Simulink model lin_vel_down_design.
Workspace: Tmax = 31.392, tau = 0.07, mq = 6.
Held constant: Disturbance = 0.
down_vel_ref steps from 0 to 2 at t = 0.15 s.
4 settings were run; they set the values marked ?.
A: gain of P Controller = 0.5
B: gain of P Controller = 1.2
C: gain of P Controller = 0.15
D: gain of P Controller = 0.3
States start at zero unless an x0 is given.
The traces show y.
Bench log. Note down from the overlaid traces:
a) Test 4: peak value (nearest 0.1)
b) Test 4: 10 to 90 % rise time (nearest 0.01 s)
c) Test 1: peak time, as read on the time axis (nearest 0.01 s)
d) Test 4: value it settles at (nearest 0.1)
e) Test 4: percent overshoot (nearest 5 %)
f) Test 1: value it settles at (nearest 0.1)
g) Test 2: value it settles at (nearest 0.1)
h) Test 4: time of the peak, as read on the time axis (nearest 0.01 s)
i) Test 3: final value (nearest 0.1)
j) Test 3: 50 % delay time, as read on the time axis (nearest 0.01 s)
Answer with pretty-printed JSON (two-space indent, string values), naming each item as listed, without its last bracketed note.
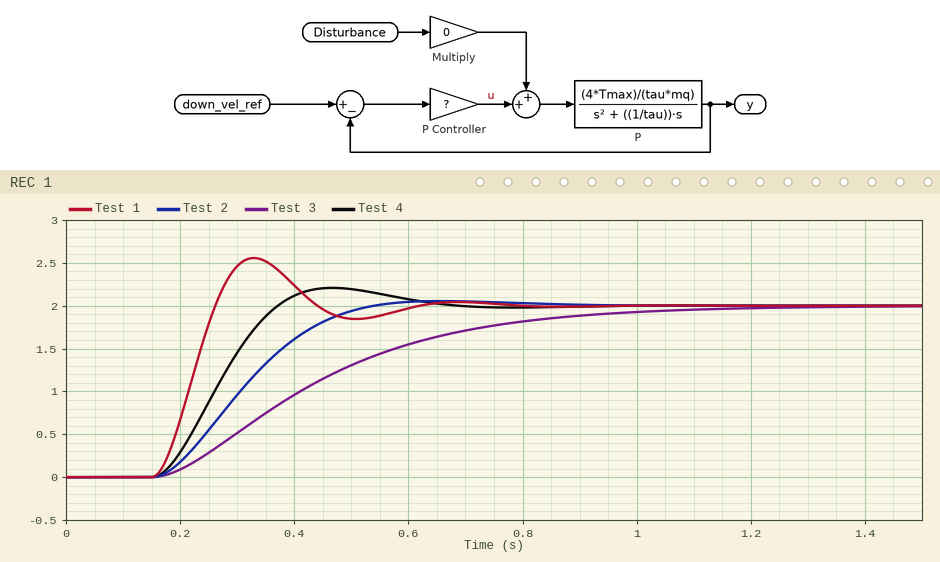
{
  "Test 4: peak value": "2.2",
  "Test 4: 10 to 90 % rise time": "0.15 s",
  "Test 1: peak time, as read on the time axis": "0.33 s",
  "Test 4: value it settles at": "2.0",
  "Test 4: percent overshoot": "10 %",
  "Test 1: value it settles at": "2.0",
  "Test 2: value it settles at": "2.0",
  "Test 4: time of the peak, as read on the time axis": "0.47 s",
  "Test 3: final value": "2.0",
  "Test 3: 50 % delay time, as read on the time axis": "0.41 s"
}
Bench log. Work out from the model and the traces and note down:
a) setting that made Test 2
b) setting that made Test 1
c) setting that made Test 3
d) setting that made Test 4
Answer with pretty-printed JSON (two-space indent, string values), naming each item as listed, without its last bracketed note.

{
  "setting that made Test 2": "D",
  "setting that made Test 1": "B",
  "setting that made Test 3": "C",
  "setting that made Test 4": "A"
}
